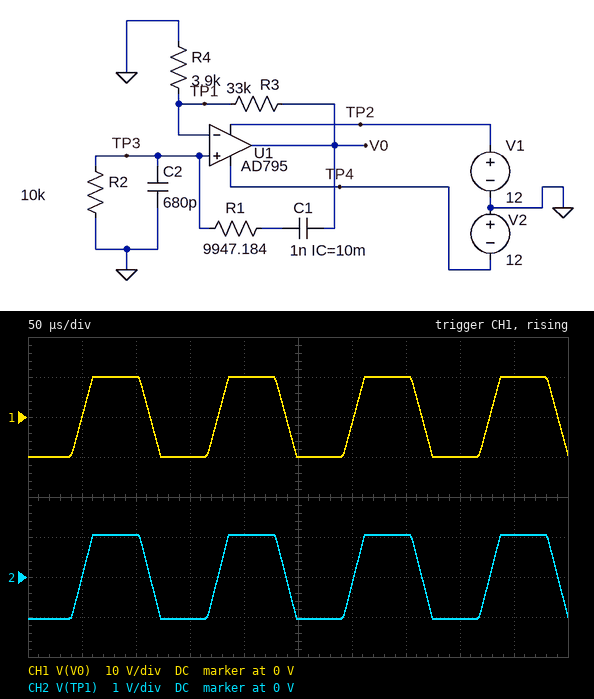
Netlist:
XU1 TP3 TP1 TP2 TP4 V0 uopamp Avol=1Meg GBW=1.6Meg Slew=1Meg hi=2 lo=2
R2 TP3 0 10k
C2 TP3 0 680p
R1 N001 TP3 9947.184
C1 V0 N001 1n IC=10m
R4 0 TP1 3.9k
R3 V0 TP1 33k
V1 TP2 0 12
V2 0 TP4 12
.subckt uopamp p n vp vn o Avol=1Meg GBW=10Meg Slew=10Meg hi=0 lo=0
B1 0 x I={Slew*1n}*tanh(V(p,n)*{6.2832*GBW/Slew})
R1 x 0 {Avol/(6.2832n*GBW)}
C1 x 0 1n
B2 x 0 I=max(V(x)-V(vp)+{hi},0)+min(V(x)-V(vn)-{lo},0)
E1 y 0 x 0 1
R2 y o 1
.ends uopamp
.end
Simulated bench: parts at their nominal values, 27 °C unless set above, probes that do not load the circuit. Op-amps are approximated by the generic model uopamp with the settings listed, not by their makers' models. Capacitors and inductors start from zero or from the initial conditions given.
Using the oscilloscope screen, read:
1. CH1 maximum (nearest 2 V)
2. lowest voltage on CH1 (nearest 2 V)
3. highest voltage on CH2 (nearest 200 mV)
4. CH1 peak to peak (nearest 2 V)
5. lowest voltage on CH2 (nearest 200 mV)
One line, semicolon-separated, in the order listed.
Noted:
10 V; -10 V; 1.0 V; 20 V; -1.0 V
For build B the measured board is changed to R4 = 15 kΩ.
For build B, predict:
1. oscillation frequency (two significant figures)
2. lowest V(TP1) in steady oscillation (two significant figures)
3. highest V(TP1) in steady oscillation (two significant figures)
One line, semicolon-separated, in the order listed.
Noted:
15 kHz; -3.1 V; 3.1 V
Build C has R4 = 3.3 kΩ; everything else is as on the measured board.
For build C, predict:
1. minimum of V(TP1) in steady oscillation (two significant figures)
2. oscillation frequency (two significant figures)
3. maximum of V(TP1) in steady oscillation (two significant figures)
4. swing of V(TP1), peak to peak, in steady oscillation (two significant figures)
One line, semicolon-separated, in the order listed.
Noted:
-910 mV; 7.5 kHz; 910 mV; 1.8 V
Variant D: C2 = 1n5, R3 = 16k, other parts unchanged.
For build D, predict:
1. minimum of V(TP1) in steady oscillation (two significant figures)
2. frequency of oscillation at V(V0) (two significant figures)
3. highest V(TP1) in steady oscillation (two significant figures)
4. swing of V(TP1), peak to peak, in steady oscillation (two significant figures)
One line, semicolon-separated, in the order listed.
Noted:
-2.0 V; 9.8 kHz; 2.0 V; 3.9 V
